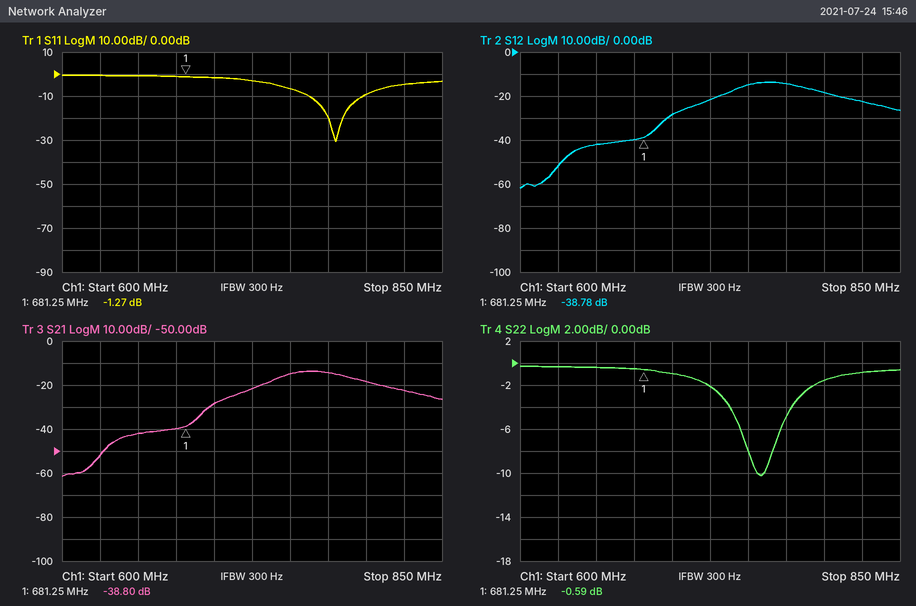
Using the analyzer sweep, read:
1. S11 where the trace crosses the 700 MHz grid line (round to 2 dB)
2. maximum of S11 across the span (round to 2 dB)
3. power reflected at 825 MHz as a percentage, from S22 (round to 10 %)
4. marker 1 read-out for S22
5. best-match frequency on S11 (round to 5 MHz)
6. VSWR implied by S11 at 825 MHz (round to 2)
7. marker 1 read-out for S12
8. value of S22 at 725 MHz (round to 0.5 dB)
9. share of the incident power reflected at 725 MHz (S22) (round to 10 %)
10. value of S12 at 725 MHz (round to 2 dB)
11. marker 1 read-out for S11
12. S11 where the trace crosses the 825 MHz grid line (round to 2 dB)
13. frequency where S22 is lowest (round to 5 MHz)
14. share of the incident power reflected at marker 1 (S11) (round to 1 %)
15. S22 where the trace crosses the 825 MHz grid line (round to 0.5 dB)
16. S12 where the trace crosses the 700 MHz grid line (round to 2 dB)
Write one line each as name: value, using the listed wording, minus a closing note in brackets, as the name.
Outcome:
S11 where the trace crosses the 700 MHz grid line: -2 dB
maximum of S11 across the span: 0 dB
power reflected at 825 MHz as a percentage, from S22: 80 %
marker 1 read-out for S22: -0.59 dB
best-match frequency on S11: 780 MHz
VSWR implied by S11 at 825 MHz: 4
marker 1 read-out for S12: -38.78 dB
value of S22 at 725 MHz: -2.0 dB
share of the incident power reflected at 725 MHz (S22): 60 %
value of S12 at 725 MHz: -22 dB
marker 1 read-out for S11: -1.27 dB
S11 where the trace crosses the 825 MHz grid line: -4 dB
frequency where S22 is lowest: 760 MHz
share of the incident power reflected at marker 1 (S11): 75 %
S22 where the trace crosses the 825 MHz grid line: -1.0 dB
S12 where the trace crosses the 700 MHz grid line: -28 dB
